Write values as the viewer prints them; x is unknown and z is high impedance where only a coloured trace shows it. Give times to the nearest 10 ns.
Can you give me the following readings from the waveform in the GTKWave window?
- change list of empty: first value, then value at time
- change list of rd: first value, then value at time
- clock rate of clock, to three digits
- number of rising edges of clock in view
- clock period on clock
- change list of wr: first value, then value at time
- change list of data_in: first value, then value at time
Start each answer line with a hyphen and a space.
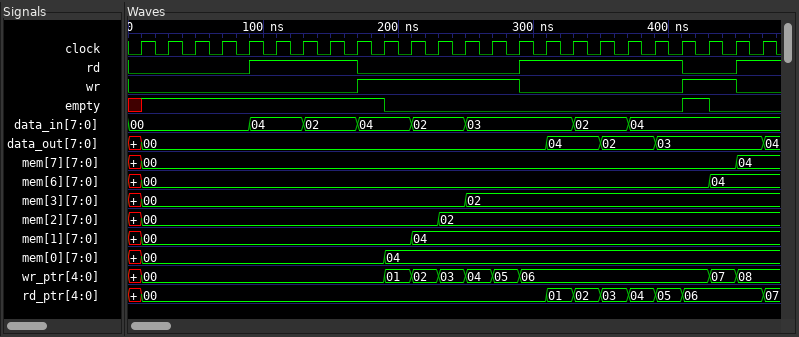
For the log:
- x, 1 at 10 ns, 0 at 190 ns, 1 at 410 ns, 0 at 430 ns
- 0, 1 at 90 ns, 0 at 170 ns, 1 at 290 ns, 0 at 410 ns, 1 at 450 ns
- 50.0 MHz
- 24
- 20 ns
- 0, 1 at 170 ns, 0 at 290 ns, 1 at 410 ns, 0 at 450 ns
- 00, 04 at 90 ns, 02 at 130 ns, 04 at 170 ns, 02 at 210 ns, 03 at 250 ns, 02 at 330 ns, 04 at 370 ns
